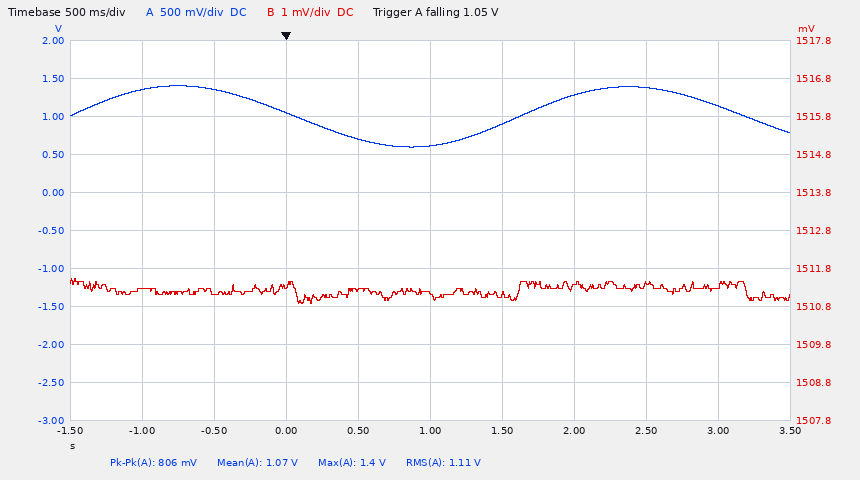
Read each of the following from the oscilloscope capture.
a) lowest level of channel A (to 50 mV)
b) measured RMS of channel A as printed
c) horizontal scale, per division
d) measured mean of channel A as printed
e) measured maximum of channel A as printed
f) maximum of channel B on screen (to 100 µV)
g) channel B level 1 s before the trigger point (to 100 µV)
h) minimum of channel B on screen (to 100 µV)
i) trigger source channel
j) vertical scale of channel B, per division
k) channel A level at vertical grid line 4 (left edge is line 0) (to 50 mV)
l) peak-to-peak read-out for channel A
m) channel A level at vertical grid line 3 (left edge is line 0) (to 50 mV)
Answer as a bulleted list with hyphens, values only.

- 600 mV
- 1.11 V
- 500 ms
- 1.07 V
- 1.4 V
- 1.5115 V
- 1.5113 V
- 1.5109 V
- channel A
- 1 mV
- 700 mV
- 806 mV
- 1.05 V
